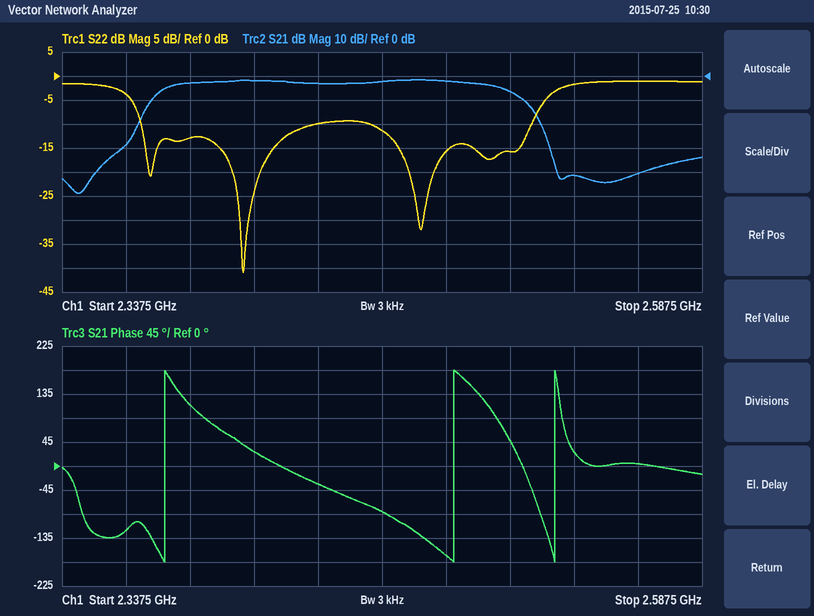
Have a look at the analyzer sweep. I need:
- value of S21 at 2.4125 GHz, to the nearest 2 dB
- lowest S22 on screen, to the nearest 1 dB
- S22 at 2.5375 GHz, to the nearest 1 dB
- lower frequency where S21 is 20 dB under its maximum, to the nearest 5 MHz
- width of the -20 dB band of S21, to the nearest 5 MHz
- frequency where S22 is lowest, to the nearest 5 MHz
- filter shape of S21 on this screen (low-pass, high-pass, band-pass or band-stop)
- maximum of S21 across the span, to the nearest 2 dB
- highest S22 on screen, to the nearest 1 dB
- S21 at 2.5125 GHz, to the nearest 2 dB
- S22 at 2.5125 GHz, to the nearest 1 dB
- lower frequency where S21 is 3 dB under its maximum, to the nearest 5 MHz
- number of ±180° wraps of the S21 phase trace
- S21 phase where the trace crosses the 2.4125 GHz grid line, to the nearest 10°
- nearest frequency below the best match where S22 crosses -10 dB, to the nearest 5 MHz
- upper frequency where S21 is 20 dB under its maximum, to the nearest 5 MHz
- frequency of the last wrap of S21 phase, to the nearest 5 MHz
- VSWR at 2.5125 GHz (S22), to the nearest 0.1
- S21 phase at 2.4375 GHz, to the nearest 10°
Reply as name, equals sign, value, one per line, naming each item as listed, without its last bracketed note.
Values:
value of S21 at 2.4125 GHz, to the nearest 2 dB = -2 dB
lowest S22 on screen, to the nearest 1 dB = -41 dB
S22 at 2.5375 GHz, to the nearest 1 dB = -2 dB
lower frequency where S21 is 20 dB under its maximum, to the nearest 5 MHz = 2.365 GHz
width of the -20 dB band of S21, to the nearest 5 MHz = 160 MHz
frequency where S22 is lowest, to the nearest 5 MHz = 2.410 GHz
filter shape of S21 on this screen = band-pass
maximum of S21 across the span, to the nearest 2 dB = -2 dB
highest S22 on screen, to the nearest 1 dB = -1 dB
S21 at 2.5125 GHz, to the nearest 2 dB = -6 dB
S22 at 2.5125 GHz, to the nearest 1 dB = -16 dB
lower frequency where S21 is 3 dB under its maximum, to the nearest 5 MHz = 2.380 GHz
number of ±180° wraps of the S21 phase trace = 3
S21 phase where the trace crosses the 2.4125 GHz grid line, to the nearest 10° = 30°
nearest frequency below the best match where S22 crosses -10 dB, to the nearest 5 MHz = 2.370 GHz
upper frequency where S21 is 20 dB under its maximum, to the nearest 5 MHz = 2.525 GHz
frequency of the last wrap of S21 phase, to the nearest 5 MHz = 2.530 GHz
VSWR at 2.5125 GHz (S22), to the nearest 0.1 = 1.4
S21 phase at 2.4375 GHz, to the nearest 10° = -30°
